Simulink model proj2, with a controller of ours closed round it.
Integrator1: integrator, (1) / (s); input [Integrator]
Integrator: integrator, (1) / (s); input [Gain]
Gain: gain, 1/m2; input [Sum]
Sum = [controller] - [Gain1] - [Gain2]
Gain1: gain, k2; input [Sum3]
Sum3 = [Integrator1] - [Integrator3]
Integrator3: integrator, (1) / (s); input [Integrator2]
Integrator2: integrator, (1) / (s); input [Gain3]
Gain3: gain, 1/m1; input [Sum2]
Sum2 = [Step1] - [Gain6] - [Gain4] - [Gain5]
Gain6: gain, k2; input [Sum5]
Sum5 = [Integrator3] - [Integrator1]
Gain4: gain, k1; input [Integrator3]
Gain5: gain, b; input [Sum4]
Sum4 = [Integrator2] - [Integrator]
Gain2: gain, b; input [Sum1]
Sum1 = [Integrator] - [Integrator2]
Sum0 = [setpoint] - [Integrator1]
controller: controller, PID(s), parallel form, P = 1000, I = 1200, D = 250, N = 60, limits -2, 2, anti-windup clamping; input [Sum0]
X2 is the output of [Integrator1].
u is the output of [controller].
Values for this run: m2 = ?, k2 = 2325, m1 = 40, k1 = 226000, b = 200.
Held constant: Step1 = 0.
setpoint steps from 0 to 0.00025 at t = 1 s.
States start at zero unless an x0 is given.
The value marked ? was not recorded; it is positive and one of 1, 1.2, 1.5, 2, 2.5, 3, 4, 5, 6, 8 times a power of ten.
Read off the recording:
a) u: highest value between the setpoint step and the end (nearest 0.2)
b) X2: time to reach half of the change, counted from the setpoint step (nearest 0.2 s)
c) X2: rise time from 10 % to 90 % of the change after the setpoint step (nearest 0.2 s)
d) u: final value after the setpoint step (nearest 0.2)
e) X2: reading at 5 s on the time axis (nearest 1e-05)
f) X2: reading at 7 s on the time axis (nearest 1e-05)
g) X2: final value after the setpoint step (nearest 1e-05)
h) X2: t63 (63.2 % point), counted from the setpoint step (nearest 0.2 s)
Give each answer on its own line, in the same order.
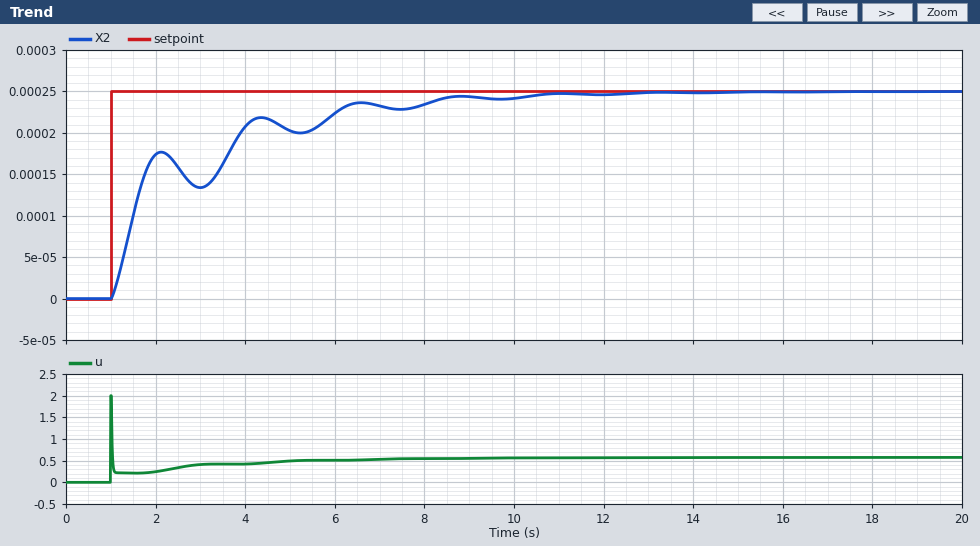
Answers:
2.0
0.6 s
4.8 s
0.6
0.00020
0.00023
0.00025
0.8 s
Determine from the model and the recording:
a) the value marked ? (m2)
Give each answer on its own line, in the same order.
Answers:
400
